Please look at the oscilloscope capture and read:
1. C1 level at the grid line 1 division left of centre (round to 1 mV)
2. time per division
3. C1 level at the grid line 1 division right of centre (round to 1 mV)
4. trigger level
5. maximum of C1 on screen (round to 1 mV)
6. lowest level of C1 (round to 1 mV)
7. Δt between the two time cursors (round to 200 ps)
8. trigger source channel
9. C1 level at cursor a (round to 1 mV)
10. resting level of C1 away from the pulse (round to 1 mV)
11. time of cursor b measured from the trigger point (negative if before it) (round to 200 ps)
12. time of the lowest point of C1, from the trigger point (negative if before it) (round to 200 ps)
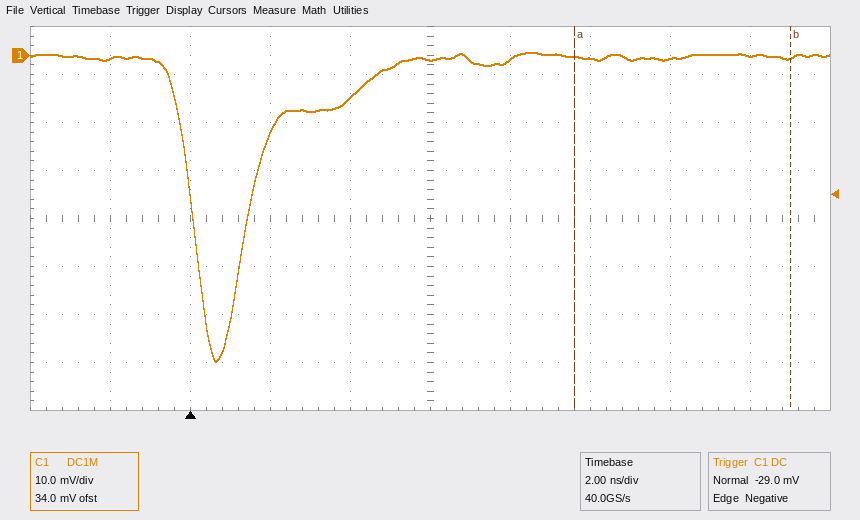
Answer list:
-9 mV
2 ns
-1 mV
-29.0 mV
1 mV
-64 mV
5.4 ns
C1
0 mV
0 mV
+15.0 ns
+600 ps
